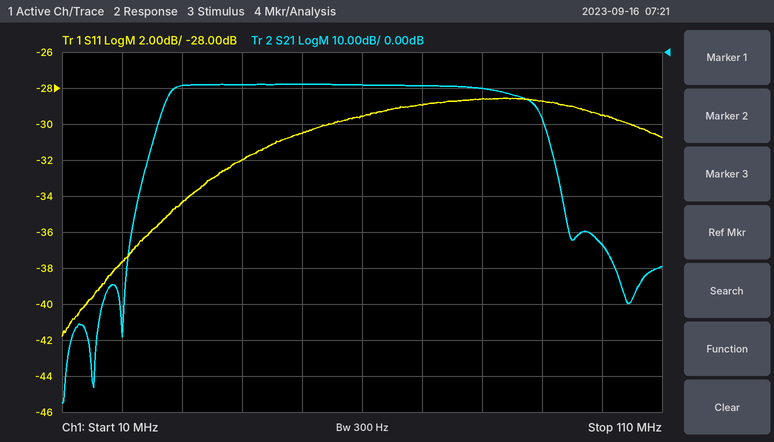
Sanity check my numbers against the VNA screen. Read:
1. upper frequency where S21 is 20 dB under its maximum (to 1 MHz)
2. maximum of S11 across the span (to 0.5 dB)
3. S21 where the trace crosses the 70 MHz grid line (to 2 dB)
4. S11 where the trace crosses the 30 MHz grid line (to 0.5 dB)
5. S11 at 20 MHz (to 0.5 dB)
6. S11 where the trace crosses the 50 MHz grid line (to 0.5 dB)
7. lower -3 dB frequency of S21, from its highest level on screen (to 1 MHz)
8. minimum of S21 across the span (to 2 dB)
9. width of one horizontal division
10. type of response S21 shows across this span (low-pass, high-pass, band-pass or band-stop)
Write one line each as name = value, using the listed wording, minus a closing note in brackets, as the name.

upper frequency where S21 is 20 dB under its maximum = 92 MHz
maximum of S11 across the span = -28.5 dB
S21 where the trace crosses the 70 MHz grid line = -10 dB
S11 where the trace crosses the 30 MHz grid line = -34.5 dB
S11 at 20 MHz = -37.5 dB
S11 where the trace crosses the 50 MHz grid line = -30.5 dB
lower -3 dB frequency of S21, from its highest level on screen = 28 MHz
minimum of S21 across the span = -98 dB
width of one horizontal division = 10 MHz
type of response S21 shows across this span = band-pass
